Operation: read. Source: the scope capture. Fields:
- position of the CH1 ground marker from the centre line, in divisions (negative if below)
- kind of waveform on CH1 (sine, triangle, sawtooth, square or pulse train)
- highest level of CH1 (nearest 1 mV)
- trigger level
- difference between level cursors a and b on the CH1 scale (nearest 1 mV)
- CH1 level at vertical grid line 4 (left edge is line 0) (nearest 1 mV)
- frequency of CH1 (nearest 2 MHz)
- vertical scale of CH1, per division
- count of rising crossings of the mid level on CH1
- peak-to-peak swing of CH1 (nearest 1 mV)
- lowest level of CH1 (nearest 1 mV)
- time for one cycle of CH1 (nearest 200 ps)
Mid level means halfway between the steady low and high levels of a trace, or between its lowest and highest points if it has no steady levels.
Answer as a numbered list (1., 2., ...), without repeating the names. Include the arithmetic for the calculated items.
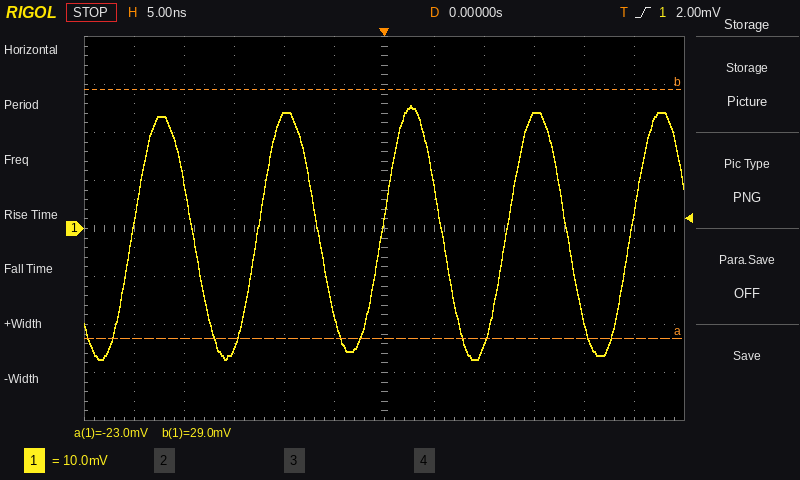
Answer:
1. 0.0 div
2. sine
3. 26 mV
4. 2.00 mV
5. 52 mV
6. 24 mV
7. 1 / 12.4 ns ≈ 80.6 MHz, so 80 MHz to the nearest 2 MHz
8. 10 mV
9. 5
10. 26 mV − (-27 mV) = 53 mV
11. -27 mV
12. 12.4 ns
